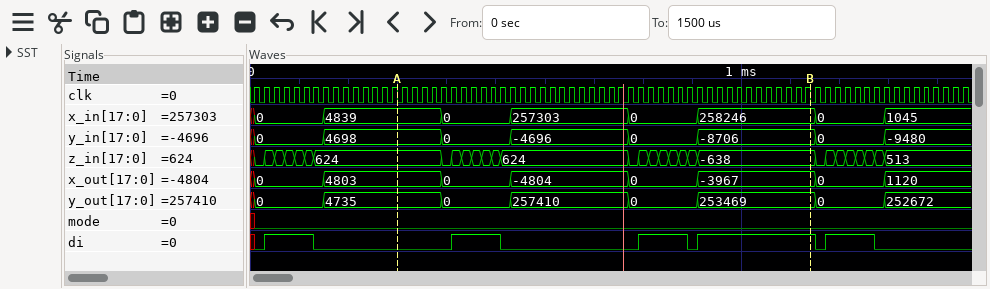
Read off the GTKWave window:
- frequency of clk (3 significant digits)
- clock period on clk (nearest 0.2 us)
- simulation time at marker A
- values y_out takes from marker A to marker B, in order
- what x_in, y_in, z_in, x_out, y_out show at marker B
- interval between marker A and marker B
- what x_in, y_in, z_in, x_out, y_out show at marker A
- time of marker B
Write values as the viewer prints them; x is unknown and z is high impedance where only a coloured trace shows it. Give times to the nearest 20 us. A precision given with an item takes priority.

50.0 kHz
20 us
300 us
4735, 0, 257410, 0, 253469
x_in=258246, y_in=-8706, z_in=-638, x_out=-3967, y_out=253469
840 us
x_in=4839, y_in=4698, z_in=624, x_out=4803, y_out=4735
1140 us
